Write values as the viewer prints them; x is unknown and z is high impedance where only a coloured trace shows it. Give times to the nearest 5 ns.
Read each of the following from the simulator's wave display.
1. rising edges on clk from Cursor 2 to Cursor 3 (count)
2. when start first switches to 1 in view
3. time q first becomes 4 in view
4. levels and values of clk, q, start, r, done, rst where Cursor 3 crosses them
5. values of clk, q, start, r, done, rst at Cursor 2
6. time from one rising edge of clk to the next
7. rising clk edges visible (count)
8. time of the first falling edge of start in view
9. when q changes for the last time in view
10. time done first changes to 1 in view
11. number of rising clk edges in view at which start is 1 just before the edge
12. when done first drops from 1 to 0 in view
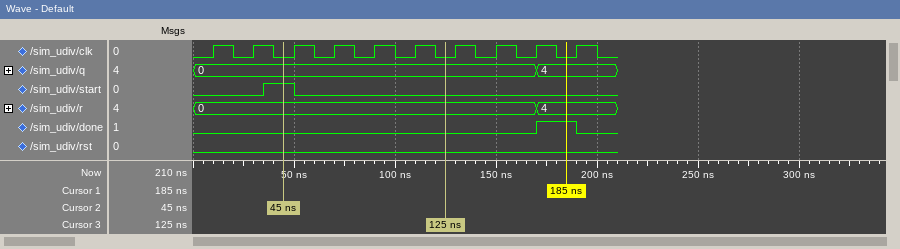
4
35 ns
170 ns
clk=0, q=0, start=0, r=0, done=0, rst=0
clk=0, q=0, start=1, r=0, done=0, rst=0
20 ns
10
50 ns
170 ns
170 ns
1
190 ns
